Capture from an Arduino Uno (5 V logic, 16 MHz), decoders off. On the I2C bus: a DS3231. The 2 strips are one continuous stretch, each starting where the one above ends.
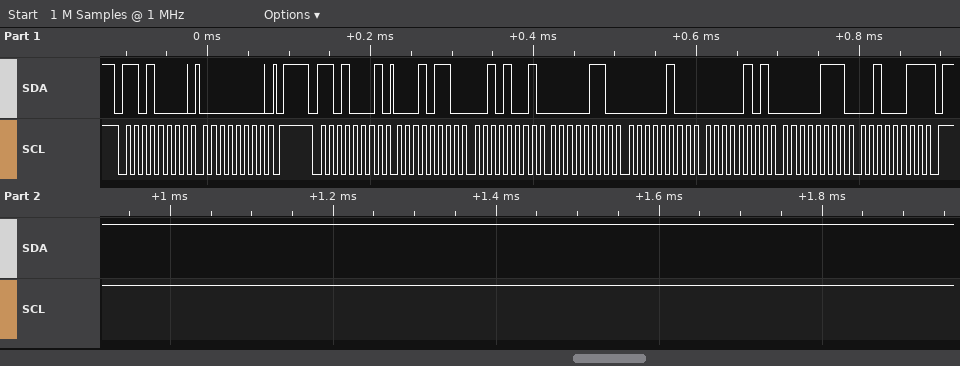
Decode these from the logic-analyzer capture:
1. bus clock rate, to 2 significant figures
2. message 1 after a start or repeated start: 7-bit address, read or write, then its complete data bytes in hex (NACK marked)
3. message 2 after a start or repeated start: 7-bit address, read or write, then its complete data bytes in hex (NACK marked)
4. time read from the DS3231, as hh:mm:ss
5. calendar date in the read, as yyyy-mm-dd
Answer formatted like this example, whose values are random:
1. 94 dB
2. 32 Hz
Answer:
1. 100 kHz
2. 0x68 write: 00
3. 0x68 read: 16 29 06 04 05 07 23 NACK
4. 06:29:16
5. 2023-07-05
